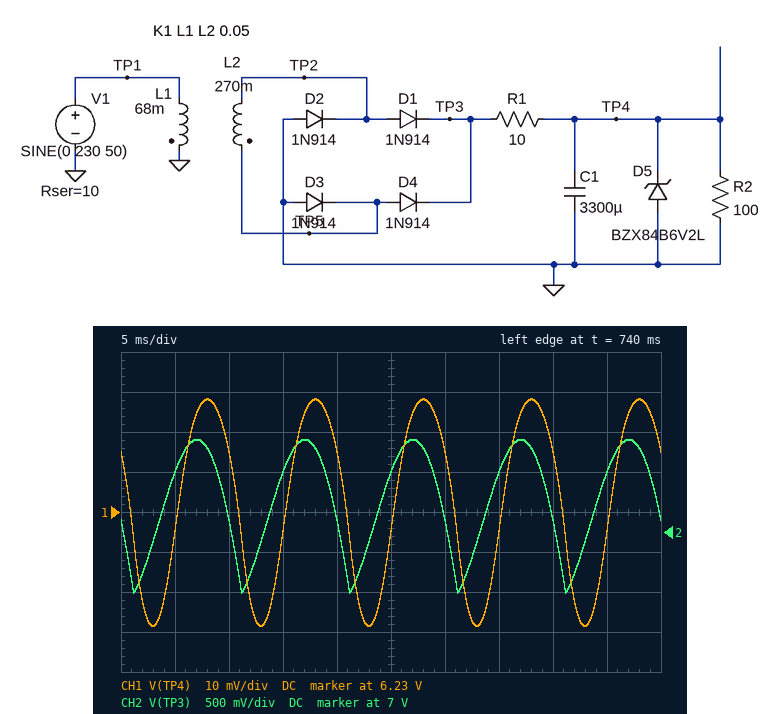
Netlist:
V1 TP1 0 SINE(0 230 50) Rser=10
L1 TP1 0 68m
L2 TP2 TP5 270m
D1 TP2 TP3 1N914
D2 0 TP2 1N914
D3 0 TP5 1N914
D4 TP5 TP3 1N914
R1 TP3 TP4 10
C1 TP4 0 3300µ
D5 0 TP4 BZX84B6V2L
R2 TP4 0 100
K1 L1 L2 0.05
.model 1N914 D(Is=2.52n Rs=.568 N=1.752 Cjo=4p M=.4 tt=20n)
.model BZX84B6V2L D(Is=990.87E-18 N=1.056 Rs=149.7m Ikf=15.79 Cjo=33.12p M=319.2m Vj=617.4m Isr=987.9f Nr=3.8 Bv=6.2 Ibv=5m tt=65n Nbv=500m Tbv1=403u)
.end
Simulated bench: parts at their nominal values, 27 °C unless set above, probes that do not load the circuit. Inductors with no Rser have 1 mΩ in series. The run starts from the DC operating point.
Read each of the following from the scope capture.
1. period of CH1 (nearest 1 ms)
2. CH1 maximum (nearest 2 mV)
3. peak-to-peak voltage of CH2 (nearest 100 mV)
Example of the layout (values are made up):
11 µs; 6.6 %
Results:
10 ms; 6.258 V; 1.9 V
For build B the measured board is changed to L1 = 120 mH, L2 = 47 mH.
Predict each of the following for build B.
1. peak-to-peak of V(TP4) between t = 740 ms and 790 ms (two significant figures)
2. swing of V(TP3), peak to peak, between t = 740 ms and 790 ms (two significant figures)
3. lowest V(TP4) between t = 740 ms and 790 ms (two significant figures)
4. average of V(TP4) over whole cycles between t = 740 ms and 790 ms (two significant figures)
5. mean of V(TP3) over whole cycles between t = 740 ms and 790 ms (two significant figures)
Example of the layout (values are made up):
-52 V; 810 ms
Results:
47 mV; 890 mV; 3.4 V; 3.5 V; 3.8 V
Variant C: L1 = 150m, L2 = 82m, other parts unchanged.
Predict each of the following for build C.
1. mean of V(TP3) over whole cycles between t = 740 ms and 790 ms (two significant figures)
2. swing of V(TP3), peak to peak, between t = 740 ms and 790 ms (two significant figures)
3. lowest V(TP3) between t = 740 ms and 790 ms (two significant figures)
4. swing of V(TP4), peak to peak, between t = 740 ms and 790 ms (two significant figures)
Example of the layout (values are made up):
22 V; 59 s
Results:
4.4 V; 910 mV; 4.0 V; 48 mV
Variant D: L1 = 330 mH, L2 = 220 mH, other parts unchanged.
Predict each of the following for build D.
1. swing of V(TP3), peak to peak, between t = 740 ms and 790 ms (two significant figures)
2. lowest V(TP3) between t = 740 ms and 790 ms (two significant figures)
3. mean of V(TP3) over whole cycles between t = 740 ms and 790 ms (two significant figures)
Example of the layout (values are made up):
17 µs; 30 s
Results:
690 mV; 3.7 V; 4.0 V
